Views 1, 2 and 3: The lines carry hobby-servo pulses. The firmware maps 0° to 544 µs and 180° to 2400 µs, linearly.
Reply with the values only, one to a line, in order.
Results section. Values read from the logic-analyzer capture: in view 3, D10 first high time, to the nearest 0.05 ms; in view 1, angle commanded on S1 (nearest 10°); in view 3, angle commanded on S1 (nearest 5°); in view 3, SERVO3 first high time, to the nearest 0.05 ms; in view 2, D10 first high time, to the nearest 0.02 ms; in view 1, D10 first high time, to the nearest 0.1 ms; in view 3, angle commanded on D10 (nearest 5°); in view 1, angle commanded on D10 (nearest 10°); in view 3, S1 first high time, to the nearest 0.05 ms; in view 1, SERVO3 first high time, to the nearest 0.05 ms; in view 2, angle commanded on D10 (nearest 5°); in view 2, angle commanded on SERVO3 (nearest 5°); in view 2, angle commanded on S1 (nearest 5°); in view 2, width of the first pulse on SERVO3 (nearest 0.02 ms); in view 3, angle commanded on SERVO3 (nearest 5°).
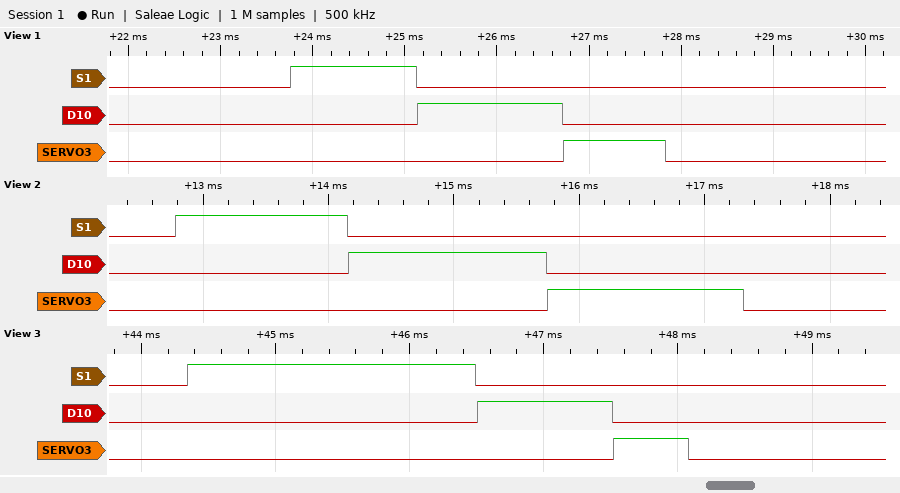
1.00 ms
80°
155°
0.55 ms
1.58 ms
1.6 ms
45°
100°
2.15 ms
1.10 ms
100°
100°
80°
1.56 ms
0°
